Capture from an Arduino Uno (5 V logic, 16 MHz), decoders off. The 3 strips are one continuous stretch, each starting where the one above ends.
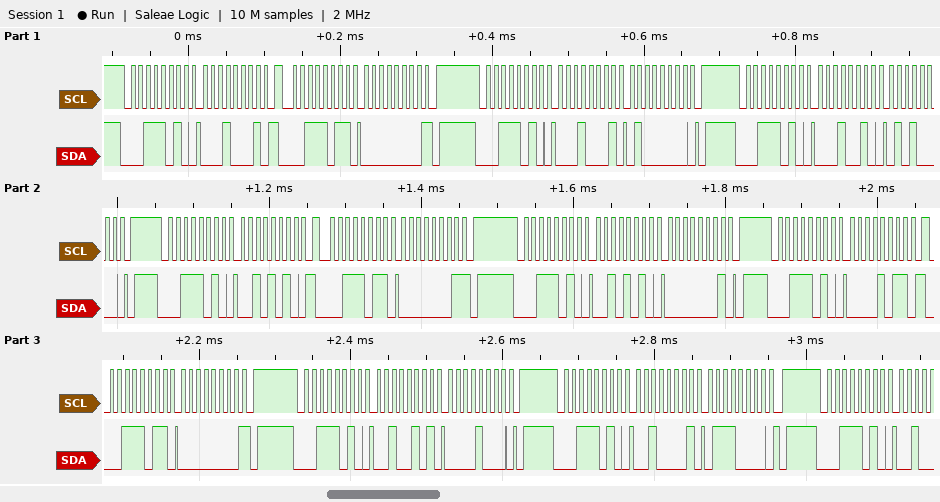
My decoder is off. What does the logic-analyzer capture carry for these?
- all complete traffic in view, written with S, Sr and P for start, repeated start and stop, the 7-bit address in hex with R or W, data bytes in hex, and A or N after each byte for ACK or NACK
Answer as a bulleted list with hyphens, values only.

- S 1DW A 11 A Sr 1DR A 00 N P S 1DW A 11 A 40 A P S 1DW A 12 A 50 A P S 1DW A 2A A Sr 1DR A 01 N P S 1DW A 2A A 01 A P S 1DW A 0B A Sr 1DR A 00 N P S 1DW A 25 A 08 A P S 1DW A 21 A 70 A P S 1DW A
